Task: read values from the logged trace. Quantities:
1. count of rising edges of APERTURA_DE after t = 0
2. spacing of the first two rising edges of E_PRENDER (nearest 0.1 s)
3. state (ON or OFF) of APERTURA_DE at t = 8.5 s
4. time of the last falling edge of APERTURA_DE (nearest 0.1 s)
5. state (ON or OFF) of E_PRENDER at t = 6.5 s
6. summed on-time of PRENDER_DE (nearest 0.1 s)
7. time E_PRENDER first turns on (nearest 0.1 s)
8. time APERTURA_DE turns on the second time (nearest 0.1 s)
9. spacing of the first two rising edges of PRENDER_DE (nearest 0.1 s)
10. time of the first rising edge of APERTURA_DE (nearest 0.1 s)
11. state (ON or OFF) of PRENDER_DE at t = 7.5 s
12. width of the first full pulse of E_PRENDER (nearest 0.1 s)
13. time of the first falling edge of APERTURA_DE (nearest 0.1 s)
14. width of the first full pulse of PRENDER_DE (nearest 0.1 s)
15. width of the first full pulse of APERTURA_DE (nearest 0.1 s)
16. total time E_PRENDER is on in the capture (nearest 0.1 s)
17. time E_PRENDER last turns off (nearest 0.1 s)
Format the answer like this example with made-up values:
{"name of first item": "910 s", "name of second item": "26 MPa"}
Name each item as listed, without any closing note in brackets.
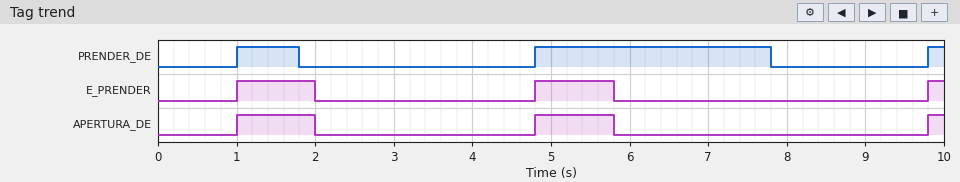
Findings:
{"count of rising edges of APERTURA_DE after t = 0": "3", "spacing of the first two rising edges of E_PRENDER": "3.8 s", "state (ON or OFF) of APERTURA_DE at t = 8.5 s": "OFF", "time of the last falling edge of APERTURA_DE": "5.8 s", "state (ON or OFF) of E_PRENDER at t = 6.5 s": "OFF", "summed on-time of PRENDER_DE": "4.0 s", "time E_PRENDER first turns on": "1.0 s", "time APERTURA_DE turns on the second time": "4.8 s", "spacing of the first two rising edges of PRENDER_DE": "3.8 s", "time of the first rising edge of APERTURA_DE": "1.0 s", "state (ON or OFF) of PRENDER_DE at t = 7.5 s": "ON", "width of the first full pulse of E_PRENDER": "1.0 s", "time of the first falling edge of APERTURA_DE": "2.0 s", "width of the first full pulse of PRENDER_DE": "0.8 s", "width of the first full pulse of APERTURA_DE": "1.0 s", "total time E_PRENDER is on in the capture": "2.2 s", "time E_PRENDER last turns off": "5.8 s"}
